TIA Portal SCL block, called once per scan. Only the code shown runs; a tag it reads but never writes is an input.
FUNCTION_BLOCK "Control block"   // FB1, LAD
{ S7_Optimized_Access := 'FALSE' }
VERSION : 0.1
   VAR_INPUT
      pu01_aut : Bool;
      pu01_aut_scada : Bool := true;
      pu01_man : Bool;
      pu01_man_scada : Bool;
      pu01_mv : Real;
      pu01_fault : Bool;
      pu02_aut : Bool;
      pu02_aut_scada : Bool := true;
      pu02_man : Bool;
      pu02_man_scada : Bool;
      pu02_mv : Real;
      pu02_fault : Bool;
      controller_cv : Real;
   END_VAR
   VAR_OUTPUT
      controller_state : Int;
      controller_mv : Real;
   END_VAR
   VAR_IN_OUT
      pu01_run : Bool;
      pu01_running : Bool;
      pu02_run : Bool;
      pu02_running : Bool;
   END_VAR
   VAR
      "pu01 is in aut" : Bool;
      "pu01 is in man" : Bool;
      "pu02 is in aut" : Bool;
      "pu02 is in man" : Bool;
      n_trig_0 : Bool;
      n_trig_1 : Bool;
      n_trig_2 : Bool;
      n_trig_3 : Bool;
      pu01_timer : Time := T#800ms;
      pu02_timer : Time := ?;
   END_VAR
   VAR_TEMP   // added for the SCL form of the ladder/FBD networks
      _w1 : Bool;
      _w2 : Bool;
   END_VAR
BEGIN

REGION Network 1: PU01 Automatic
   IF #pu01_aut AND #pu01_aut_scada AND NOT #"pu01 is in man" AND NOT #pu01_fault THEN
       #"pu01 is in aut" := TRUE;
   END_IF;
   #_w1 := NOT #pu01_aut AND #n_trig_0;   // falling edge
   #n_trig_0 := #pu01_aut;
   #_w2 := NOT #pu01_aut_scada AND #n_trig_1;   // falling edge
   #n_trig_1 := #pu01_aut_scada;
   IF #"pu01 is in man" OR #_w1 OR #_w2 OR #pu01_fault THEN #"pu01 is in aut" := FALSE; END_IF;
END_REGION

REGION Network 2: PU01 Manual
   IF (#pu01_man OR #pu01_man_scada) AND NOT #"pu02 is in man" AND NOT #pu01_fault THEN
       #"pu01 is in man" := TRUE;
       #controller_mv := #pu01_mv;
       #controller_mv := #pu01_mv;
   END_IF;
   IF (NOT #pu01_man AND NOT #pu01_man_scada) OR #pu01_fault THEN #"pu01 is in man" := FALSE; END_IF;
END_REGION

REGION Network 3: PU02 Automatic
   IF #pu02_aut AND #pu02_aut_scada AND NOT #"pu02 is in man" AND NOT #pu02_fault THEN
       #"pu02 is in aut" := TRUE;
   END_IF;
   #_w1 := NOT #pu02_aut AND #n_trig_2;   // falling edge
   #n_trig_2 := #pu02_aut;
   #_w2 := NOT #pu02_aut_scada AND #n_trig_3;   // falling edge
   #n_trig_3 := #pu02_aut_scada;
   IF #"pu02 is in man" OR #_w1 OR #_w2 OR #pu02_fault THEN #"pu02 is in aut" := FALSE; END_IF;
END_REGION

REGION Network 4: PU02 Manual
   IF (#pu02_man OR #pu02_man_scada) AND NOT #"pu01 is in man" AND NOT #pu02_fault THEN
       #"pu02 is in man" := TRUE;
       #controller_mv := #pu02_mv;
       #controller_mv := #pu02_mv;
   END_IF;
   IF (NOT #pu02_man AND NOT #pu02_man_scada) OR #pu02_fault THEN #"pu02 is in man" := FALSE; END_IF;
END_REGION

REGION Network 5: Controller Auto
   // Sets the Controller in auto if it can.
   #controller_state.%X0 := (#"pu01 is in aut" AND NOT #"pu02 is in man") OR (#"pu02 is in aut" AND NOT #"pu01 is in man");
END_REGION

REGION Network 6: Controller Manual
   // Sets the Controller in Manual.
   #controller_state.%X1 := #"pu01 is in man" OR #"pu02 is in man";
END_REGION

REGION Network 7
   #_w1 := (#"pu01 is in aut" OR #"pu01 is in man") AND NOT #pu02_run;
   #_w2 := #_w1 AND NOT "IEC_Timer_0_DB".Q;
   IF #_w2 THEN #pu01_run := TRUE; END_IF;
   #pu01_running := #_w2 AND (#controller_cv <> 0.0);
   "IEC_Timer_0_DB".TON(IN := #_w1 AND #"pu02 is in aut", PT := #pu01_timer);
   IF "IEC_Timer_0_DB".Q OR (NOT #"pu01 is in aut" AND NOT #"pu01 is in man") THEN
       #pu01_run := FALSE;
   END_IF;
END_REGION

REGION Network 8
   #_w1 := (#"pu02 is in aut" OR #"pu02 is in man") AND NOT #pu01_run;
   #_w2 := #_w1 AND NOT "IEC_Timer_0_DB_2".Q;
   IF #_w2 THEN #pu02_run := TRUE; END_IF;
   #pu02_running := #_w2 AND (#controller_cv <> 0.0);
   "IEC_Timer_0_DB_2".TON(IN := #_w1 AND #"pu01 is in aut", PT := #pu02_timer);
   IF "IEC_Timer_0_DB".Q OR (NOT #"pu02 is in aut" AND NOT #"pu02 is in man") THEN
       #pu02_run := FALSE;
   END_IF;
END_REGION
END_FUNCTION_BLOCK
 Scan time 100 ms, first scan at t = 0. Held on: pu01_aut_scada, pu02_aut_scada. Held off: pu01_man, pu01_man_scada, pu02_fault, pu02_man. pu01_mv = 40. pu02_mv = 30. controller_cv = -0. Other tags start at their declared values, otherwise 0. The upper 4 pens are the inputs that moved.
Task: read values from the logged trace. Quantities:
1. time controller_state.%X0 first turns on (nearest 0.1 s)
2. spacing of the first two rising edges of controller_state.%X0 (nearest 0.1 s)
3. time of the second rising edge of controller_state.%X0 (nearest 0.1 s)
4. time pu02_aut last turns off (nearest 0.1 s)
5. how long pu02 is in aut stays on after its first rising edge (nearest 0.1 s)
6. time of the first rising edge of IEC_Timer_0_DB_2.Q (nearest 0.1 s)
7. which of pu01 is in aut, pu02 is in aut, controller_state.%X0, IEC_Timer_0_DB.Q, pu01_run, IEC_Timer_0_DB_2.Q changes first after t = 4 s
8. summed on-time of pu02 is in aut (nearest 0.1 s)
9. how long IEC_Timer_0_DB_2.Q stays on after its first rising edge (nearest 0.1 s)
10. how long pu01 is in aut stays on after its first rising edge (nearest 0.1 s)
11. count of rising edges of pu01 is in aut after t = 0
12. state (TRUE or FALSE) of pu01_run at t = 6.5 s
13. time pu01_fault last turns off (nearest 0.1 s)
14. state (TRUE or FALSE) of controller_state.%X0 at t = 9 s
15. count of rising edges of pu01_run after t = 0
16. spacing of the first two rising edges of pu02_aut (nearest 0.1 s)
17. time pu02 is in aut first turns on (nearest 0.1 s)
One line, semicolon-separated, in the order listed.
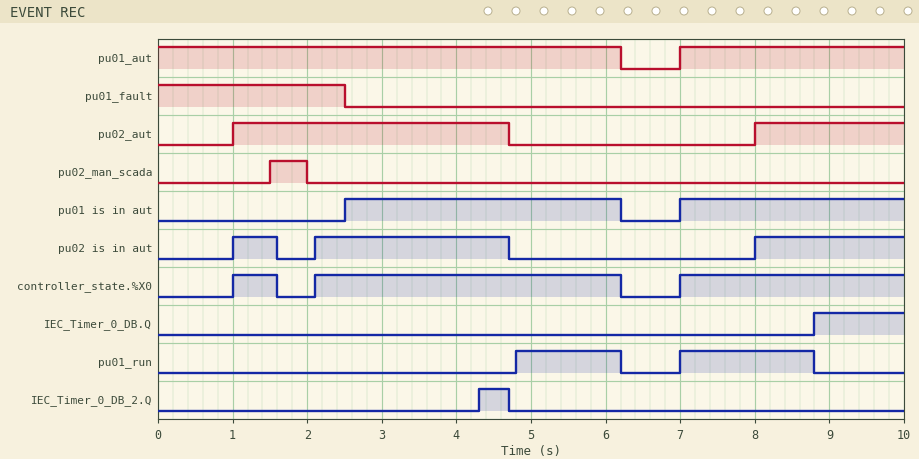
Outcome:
1.0 s; 1.1 s; 2.1 s; 4.7 s; 0.6 s; 4.3 s; IEC_Timer_0_DB_2.Q; 5.2 s; 0.4 s; 3.7 s; 2; FALSE; 2.5 s; TRUE; 2; 7.0 s; 1.0 s
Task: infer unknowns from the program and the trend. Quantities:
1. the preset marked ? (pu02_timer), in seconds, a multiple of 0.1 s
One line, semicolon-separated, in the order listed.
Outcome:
1.8 s
